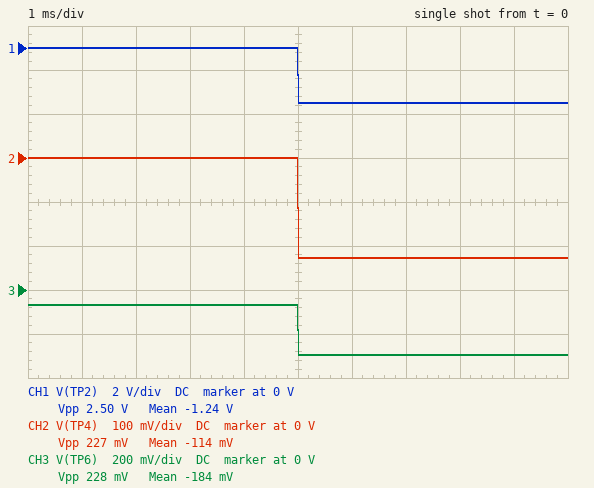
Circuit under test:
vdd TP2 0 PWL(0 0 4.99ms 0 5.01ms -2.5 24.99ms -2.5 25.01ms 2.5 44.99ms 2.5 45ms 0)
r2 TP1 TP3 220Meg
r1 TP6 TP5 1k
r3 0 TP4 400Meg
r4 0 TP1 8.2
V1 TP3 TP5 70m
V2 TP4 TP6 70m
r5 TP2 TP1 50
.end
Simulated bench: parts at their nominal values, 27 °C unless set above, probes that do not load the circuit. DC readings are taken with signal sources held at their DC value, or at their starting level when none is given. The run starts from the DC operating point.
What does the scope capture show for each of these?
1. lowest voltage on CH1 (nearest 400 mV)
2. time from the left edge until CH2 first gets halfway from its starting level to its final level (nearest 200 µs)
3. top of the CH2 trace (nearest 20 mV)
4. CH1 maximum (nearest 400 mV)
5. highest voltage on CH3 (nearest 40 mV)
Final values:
-2.4 V
5.0 ms
0 V
0 V
-80 mV
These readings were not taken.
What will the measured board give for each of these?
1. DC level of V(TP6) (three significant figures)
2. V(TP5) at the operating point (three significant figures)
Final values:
-70.0 mV
-70.0 mV
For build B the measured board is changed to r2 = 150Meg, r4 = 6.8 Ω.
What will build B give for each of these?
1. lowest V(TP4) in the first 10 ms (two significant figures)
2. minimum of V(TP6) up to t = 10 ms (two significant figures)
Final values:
-220 mV
-290 mV
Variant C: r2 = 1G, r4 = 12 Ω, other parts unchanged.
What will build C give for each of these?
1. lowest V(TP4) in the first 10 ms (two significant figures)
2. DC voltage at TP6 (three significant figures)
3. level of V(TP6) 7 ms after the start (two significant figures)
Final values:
-140 mV
-70.0 mV
-210 mV
